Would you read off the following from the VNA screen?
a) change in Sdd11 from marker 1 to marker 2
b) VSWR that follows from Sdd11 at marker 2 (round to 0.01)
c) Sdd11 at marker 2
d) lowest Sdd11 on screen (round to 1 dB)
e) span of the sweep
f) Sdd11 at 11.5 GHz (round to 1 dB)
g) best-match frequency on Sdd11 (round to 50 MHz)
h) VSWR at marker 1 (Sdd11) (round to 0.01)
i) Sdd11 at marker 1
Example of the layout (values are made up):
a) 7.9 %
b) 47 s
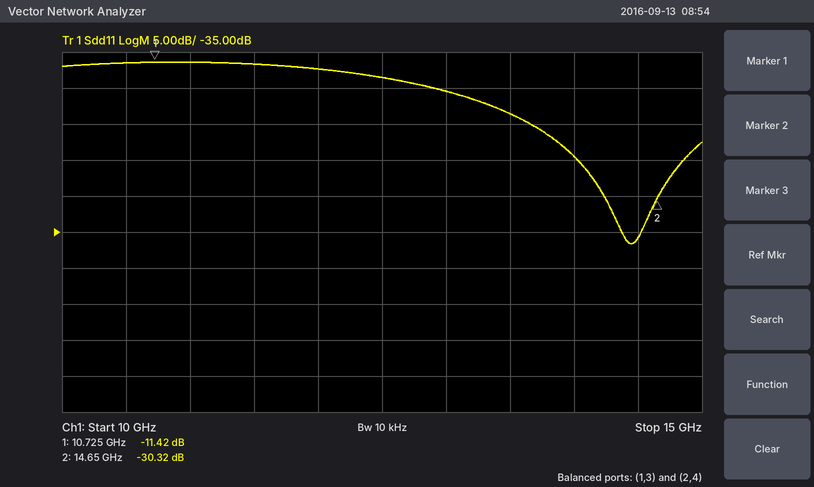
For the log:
a) -18.90 dB
b) 1.06
c) -30.32 dB
d) -37 dB
e) 5 GHz
f) -12 dB
g) 14.45 GHz
h) 1.73
i) -11.42 dB
